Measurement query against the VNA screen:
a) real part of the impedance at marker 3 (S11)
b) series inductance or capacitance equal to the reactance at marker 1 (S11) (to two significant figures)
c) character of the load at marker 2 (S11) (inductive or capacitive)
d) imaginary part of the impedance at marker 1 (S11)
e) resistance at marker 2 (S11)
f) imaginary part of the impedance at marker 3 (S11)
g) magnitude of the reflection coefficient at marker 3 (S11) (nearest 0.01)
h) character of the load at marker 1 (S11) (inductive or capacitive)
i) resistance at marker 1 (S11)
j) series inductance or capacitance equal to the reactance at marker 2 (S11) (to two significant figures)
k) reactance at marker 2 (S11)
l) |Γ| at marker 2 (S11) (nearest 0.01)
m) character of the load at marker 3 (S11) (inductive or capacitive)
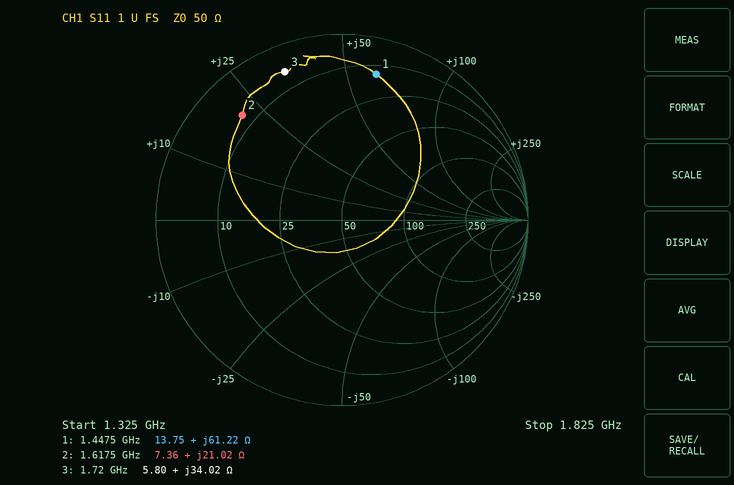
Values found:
5.80 Ω
6.7 nH
inductive
+61.22 Ω
7.36 Ω
+34.02 Ω
0.85
inductive
13.75 Ω
2.1 nH
+21.02 Ω
0.78
inductive
